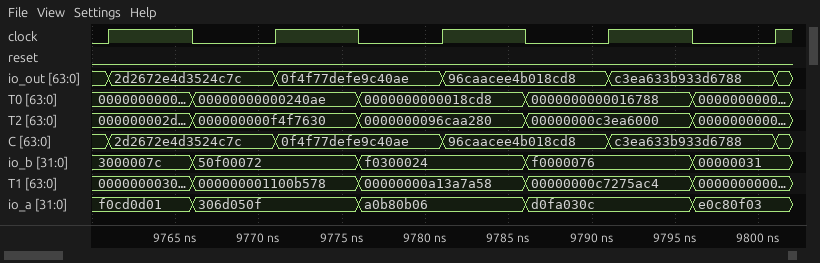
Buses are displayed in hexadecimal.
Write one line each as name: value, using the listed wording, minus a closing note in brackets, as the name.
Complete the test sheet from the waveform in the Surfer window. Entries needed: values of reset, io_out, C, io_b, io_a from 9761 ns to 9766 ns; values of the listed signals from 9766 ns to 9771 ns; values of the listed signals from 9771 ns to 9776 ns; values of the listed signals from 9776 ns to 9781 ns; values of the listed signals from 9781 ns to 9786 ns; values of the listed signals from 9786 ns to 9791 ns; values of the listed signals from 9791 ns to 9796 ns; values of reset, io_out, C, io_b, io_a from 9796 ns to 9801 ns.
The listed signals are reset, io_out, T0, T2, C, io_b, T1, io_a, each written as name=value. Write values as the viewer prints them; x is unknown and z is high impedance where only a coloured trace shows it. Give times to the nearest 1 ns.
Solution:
values of reset, io_out, C, io_b, io_a from 9761 ns to 9766 ns: reset=0, io_out=2d2672e4d3524c7c, C=2d2672e4d3524c7c, io_b=3000007c, io_a=f0cd0d01
values of the listed signals from 9766 ns to 9771 ns: reset=0, io_out=2d2672e4d3524c7c, T0=00000000000240ae, T2=000000000f4f7630, C=2d2672e4d3524c7c, io_b=50f00072, T1=000000001100b578, io_a=306d050f
values of the listed signals from 9771 ns to 9776 ns: reset=0, io_out=0f4f77defe9c40ae, T0=00000000000240ae, T2=000000000f4f7630, C=0f4f77defe9c40ae, io_b=50f00072, T1=000000001100b578, io_a=306d050f
values of the listed signals from 9776 ns to 9781 ns: reset=0, io_out=0f4f77defe9c40ae, T0=0000000000018cd8, T2=0000000096caa280, C=0f4f77defe9c40ae, io_b=f0300024, T1=00000000a13a7a58, io_a=a0b80b06
values of the listed signals from 9781 ns to 9786 ns: reset=0, io_out=96caacee4b018cd8, T0=0000000000018cd8, T2=0000000096caa280, C=96caacee4b018cd8, io_b=f0300024, T1=00000000a13a7a58, io_a=a0b80b06
values of the listed signals from 9786 ns to 9791 ns: reset=0, io_out=96caacee4b018cd8, T0=0000000000016788, T2=00000000c3ea6000, C=96caacee4b018cd8, io_b=f0000076, T1=00000000c7275ac4, io_a=d0fa030c
values of the listed signals from 9791 ns to 9796 ns: reset=0, io_out=c3ea633b933d6788, T0=0000000000016788, T2=00000000c3ea6000, C=c3ea633b933d6788, io_b=f0000076, T1=00000000c7275ac4, io_a=d0fa030c
values of reset, io_out, C, io_b, io_a from 9796 ns to 9801 ns: reset=0, io_out=c3ea633b933d6788, C=c3ea633b933d6788, io_b=00000031, io_a=e0c80f03
